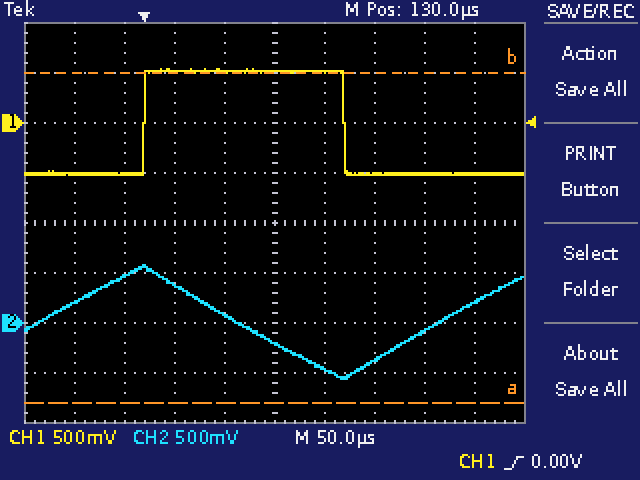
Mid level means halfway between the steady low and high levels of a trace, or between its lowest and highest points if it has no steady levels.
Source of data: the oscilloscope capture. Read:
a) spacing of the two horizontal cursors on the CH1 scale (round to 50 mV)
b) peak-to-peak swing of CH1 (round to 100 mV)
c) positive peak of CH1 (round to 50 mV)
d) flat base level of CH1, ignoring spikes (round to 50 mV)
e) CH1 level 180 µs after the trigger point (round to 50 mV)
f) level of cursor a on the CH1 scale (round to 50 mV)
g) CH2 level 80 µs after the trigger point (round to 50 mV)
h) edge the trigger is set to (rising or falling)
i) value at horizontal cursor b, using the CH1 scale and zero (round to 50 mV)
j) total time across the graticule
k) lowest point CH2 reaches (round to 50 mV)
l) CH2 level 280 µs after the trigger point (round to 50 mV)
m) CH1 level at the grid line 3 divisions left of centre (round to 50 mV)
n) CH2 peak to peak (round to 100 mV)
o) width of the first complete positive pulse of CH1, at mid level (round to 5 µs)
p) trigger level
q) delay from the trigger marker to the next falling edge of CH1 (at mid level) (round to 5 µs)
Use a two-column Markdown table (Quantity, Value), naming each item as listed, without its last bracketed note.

| Quantity | Value |
|---|---|
| spacing of the two horizontal cursors on the CH1 scale | 3.30 V |
| peak-to-peak swing of CH1 | 1.10 V |
| positive peak of CH1 | 550 mV |
| flat base level of CH1, ignoring spikes | -500 mV |
| CH1 level 180 µs after the trigger point | 500 mV |
| level of cursor a on the CH1 scale | -2.80 V |
| CH2 level 80 µs after the trigger point | 100 mV |
| edge the trigger is set to | rising |
| value at horizontal cursor b, using the CH1 scale and zero | 500 mV |
| total time across the graticule | 500 µs |
| lowest point CH2 reaches | -550 mV |
| CH2 level 280 µs after the trigger point | -100 mV |
| CH1 level at the grid line 3 divisions left of centre | -500 mV |
| CH2 peak to peak | 1.10 V |
| width of the first complete positive pulse of CH1, at mid level | 200 µs |
| trigger level | 0.00 V |
| delay from the trigger marker to the next falling edge of CH1 (at mid level) | 200 µs |
